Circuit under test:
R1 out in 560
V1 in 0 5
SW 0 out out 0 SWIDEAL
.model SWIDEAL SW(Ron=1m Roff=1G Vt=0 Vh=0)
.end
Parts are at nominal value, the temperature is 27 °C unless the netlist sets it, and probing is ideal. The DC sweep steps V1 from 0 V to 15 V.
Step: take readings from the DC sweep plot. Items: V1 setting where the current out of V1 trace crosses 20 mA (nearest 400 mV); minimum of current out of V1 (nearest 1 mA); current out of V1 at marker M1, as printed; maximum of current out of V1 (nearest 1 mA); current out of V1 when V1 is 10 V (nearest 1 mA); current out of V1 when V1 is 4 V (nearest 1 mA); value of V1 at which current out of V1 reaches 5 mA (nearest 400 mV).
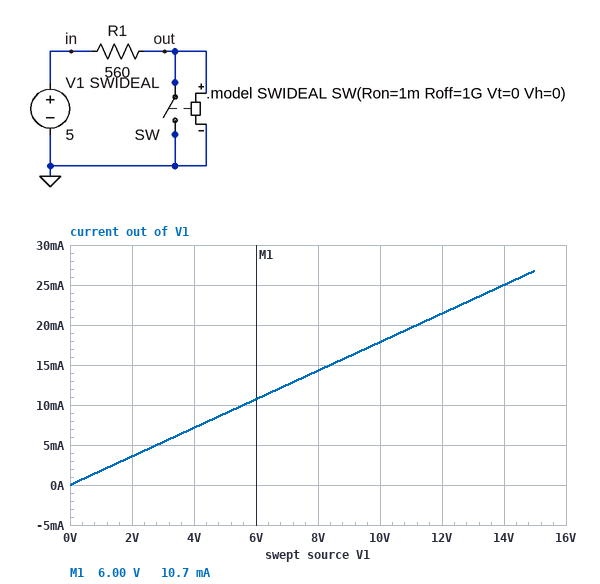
11.2 V
0 A
10.7 mA
27 mA
18 mA
7 mA
2.8 V
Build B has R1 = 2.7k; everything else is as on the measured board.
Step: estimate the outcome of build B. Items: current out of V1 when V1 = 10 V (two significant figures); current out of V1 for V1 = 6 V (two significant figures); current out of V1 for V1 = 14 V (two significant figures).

3.7 mA
2.2 mA
5.2 mA
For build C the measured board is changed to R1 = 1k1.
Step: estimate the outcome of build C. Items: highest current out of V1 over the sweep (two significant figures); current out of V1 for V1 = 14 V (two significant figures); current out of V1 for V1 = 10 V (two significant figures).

14 mA
13 mA
9.1 mA
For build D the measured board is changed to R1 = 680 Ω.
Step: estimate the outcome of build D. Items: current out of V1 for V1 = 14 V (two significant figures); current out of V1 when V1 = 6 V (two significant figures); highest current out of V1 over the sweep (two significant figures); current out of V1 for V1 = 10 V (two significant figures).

21 mA
8.8 mA
22 mA
15 mA
